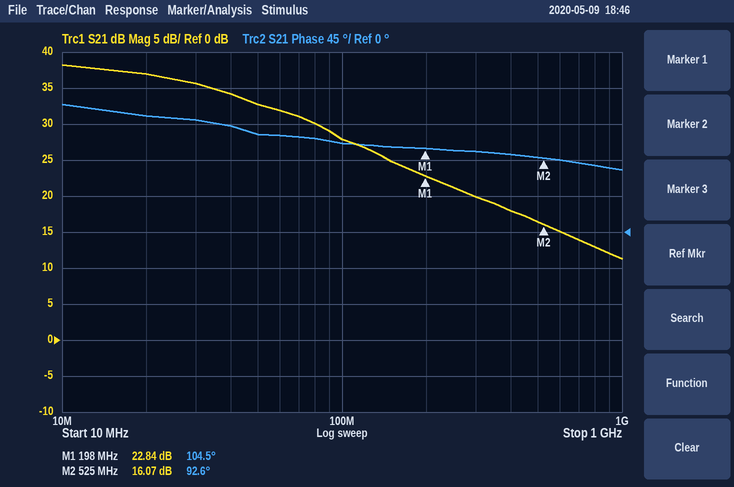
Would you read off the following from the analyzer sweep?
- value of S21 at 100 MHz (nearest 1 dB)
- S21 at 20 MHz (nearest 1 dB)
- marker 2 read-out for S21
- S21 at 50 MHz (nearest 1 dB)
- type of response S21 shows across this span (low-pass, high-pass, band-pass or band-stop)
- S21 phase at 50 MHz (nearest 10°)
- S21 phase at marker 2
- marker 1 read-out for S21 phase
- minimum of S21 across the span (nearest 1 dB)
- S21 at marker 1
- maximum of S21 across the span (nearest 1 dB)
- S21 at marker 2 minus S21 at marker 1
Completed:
28 dB
37 dB
16.07 dB
33 dB
low-pass
120°
92.6°
104.5°
11 dB
22.84 dB
38 dB
-6.77 dB
